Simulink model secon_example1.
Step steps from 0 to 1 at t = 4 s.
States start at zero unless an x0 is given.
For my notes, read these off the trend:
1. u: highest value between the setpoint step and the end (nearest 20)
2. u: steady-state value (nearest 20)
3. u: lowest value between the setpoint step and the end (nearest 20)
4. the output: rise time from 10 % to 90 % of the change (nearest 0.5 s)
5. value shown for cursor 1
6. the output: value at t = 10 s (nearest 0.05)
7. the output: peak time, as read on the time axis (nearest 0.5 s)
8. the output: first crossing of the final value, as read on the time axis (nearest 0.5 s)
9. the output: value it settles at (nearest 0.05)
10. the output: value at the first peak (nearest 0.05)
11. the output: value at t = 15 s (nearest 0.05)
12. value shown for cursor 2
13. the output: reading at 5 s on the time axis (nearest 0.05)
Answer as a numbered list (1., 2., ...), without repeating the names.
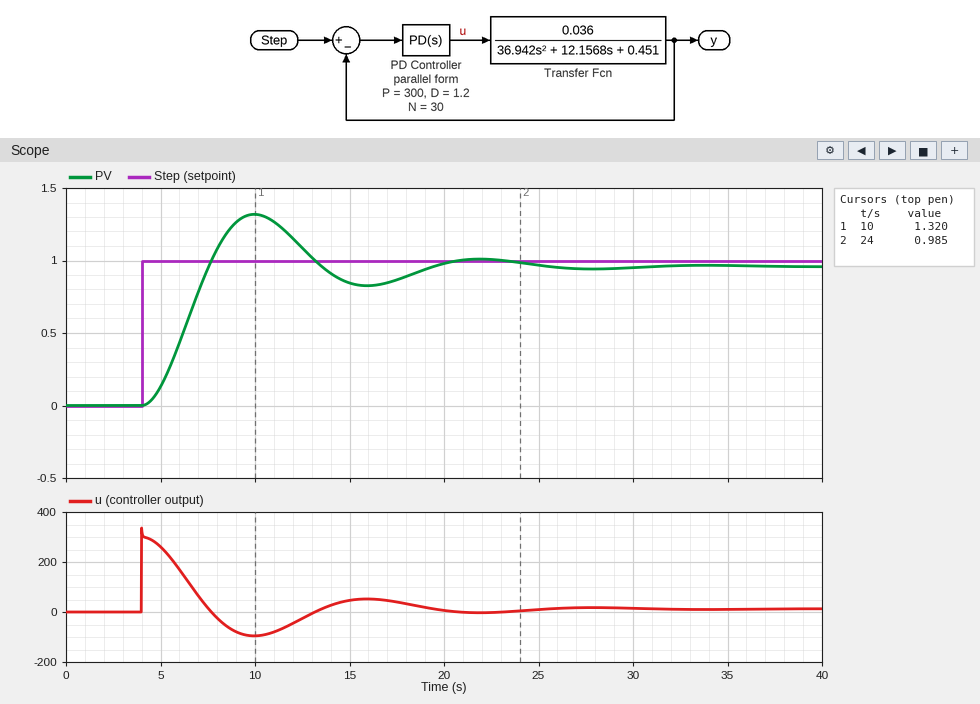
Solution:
1. 340
2. 20
3. -100
4. 2.5 s
5. 1.320
6. 1.30
7. 10.0 s
8. 7.5 s
9. 0.95
10. 1.30
11. 0.85
12. 0.985
13. 0.15
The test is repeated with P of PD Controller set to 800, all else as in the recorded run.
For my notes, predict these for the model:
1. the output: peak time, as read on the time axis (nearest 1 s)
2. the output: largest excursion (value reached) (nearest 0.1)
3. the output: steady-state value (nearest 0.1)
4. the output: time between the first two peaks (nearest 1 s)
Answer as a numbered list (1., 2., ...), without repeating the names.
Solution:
1. 8 s
2. 1.5
3. 1.0
4. 7 s
